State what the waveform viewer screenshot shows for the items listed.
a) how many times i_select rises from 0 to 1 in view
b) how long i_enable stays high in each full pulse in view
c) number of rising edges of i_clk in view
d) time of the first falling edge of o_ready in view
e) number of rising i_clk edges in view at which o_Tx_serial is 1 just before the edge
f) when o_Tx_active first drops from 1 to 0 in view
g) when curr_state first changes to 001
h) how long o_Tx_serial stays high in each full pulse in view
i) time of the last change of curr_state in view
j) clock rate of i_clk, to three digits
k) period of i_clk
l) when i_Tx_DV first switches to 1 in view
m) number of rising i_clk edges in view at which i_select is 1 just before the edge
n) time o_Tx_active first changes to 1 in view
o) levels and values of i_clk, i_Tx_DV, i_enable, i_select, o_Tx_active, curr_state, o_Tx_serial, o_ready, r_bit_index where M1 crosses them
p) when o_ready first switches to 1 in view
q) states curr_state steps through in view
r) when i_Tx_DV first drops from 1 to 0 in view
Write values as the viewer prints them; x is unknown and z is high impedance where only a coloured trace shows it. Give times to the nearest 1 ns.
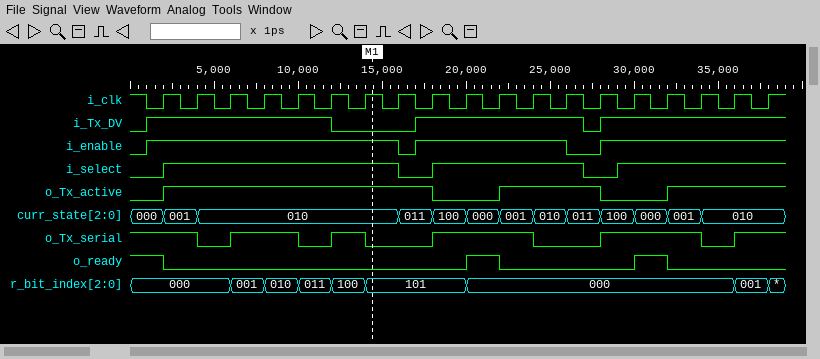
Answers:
3
15 ns, 9 ns
19
2 ns
12
18 ns
2 ns
4 ns, 2 ns, 6 ns, 6 ns
34 ns
500 MHz
2 ns
1 ns
16
2 ns
i_clk=1, i_Tx_DV=0, i_enable=1, i_select=1, o_Tx_active=1, curr_state=010, o_Tx_serial=0, o_ready=0, r_bit_index=101
20 ns
000, 001, 010, 011, 100, 000, 001, 010, 011, 100, 000, 001, 010
12 ns
